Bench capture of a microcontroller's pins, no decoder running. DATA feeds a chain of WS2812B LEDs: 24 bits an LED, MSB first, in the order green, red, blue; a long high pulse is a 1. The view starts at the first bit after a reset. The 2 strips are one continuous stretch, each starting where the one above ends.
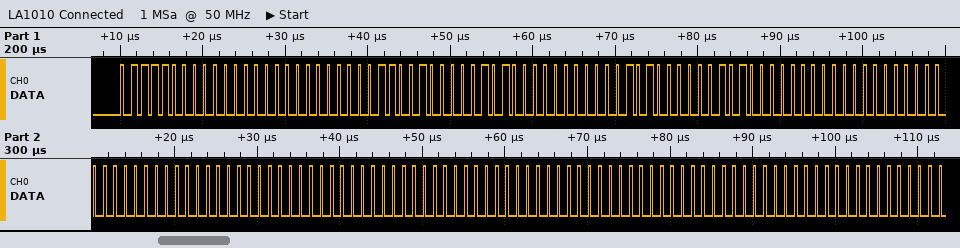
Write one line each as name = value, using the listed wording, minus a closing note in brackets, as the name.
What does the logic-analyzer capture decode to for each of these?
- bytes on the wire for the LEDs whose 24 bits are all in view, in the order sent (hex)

bytes on the wire for the LEDs whose 24 bits are all in view, in the order sent = 78 00 00 64 14 00 50 28 00 00 00 00 00 00 00 00 00 00
